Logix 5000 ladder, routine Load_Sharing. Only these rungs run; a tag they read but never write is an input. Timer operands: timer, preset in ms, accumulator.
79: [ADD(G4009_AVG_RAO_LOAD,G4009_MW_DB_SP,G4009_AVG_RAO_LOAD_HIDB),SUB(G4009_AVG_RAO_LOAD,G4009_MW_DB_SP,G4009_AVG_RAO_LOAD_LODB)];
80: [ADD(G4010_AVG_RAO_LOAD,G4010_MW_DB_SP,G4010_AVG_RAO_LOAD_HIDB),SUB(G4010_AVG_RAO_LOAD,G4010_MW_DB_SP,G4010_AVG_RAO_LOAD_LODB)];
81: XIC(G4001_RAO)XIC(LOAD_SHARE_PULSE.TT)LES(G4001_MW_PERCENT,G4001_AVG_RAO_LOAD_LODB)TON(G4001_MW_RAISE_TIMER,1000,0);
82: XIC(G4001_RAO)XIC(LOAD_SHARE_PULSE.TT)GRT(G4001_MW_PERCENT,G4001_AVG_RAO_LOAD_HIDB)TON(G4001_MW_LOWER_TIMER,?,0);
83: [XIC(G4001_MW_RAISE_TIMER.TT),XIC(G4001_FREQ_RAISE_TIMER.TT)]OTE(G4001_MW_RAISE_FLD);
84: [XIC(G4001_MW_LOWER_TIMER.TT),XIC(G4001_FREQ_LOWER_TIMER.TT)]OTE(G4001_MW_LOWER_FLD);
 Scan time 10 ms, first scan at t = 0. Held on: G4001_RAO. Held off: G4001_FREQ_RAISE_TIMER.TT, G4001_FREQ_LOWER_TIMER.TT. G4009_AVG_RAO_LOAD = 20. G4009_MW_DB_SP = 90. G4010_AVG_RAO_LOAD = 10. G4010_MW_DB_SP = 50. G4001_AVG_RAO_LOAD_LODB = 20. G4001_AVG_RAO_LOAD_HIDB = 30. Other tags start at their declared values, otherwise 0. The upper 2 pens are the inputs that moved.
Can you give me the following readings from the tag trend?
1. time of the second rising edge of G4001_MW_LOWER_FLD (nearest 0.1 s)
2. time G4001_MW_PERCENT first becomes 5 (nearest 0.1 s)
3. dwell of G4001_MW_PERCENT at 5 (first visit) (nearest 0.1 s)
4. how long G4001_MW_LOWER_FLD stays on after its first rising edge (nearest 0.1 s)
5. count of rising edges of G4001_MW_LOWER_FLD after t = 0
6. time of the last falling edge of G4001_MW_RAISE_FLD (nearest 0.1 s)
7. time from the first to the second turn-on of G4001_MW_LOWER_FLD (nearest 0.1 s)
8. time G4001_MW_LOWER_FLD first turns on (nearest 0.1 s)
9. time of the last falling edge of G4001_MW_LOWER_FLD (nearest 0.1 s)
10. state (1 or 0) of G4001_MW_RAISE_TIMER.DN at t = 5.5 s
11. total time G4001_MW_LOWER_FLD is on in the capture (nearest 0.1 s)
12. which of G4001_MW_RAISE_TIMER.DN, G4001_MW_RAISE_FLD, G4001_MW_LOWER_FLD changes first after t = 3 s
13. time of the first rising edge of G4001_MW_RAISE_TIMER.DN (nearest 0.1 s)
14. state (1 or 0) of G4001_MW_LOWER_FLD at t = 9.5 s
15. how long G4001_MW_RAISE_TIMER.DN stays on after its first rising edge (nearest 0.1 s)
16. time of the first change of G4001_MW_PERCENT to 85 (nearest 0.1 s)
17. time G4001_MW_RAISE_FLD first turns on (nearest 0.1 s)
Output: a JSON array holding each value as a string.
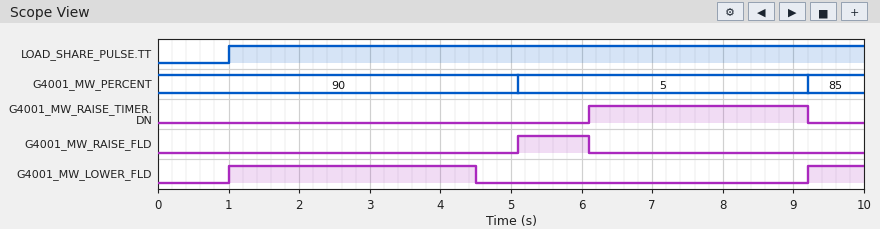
["9.2 s", "5.1 s", "4.1 s", "3.5 s", "2", "6.1 s", "8.2 s", "1.0 s", "4.5 s", "0", "4.3 s", "G4001_MW_LOWER_FLD", "6.1 s", "1", "3.1 s", "9.2 s", "5.1 s"]
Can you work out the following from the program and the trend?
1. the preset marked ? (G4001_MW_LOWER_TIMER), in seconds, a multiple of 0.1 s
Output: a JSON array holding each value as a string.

["3.5 s"]
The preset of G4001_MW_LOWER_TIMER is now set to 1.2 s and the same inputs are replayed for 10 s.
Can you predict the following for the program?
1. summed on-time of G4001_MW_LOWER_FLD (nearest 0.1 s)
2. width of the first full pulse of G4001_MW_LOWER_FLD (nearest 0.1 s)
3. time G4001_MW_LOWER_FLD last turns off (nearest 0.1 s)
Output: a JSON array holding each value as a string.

["2.0 s", "1.2 s", "2.2 s"]
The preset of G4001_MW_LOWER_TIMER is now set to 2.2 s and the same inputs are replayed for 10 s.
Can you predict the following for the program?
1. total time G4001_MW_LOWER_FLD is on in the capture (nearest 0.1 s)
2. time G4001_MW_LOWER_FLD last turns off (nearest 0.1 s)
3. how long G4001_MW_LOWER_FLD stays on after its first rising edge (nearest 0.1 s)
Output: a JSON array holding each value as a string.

["3.0 s", "3.2 s", "2.2 s"]
